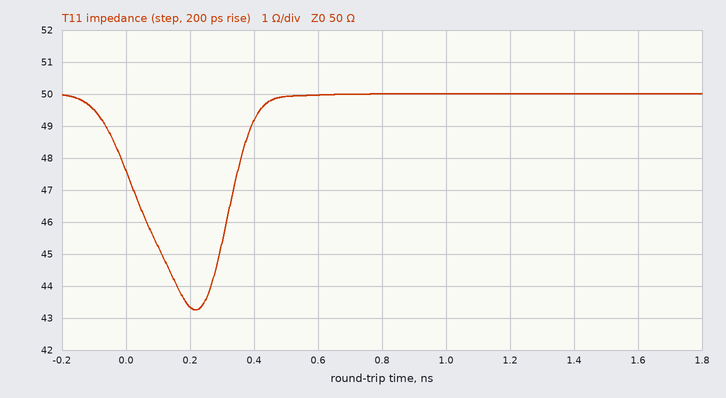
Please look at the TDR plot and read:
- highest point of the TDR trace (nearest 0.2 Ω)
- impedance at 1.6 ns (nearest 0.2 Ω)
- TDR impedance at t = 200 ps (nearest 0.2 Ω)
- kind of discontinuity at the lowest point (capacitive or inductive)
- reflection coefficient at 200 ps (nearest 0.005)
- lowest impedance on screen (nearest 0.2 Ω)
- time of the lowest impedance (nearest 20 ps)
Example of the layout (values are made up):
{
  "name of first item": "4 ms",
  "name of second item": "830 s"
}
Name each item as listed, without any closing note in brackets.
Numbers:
{
  "highest point of the TDR trace": "50.0 Ω",
  "impedance at 1.6 ns": "50.0 Ω",
  "TDR impedance at t = 200 ps": "43.4 Ω",
  "kind of discontinuity at the lowest point": "capacitive",
  "reflection coefficient at 200 ps": "-0.070",
  "lowest impedance on screen": "43.2 Ω",
  "time of the lowest impedance": "220 ps"
}
